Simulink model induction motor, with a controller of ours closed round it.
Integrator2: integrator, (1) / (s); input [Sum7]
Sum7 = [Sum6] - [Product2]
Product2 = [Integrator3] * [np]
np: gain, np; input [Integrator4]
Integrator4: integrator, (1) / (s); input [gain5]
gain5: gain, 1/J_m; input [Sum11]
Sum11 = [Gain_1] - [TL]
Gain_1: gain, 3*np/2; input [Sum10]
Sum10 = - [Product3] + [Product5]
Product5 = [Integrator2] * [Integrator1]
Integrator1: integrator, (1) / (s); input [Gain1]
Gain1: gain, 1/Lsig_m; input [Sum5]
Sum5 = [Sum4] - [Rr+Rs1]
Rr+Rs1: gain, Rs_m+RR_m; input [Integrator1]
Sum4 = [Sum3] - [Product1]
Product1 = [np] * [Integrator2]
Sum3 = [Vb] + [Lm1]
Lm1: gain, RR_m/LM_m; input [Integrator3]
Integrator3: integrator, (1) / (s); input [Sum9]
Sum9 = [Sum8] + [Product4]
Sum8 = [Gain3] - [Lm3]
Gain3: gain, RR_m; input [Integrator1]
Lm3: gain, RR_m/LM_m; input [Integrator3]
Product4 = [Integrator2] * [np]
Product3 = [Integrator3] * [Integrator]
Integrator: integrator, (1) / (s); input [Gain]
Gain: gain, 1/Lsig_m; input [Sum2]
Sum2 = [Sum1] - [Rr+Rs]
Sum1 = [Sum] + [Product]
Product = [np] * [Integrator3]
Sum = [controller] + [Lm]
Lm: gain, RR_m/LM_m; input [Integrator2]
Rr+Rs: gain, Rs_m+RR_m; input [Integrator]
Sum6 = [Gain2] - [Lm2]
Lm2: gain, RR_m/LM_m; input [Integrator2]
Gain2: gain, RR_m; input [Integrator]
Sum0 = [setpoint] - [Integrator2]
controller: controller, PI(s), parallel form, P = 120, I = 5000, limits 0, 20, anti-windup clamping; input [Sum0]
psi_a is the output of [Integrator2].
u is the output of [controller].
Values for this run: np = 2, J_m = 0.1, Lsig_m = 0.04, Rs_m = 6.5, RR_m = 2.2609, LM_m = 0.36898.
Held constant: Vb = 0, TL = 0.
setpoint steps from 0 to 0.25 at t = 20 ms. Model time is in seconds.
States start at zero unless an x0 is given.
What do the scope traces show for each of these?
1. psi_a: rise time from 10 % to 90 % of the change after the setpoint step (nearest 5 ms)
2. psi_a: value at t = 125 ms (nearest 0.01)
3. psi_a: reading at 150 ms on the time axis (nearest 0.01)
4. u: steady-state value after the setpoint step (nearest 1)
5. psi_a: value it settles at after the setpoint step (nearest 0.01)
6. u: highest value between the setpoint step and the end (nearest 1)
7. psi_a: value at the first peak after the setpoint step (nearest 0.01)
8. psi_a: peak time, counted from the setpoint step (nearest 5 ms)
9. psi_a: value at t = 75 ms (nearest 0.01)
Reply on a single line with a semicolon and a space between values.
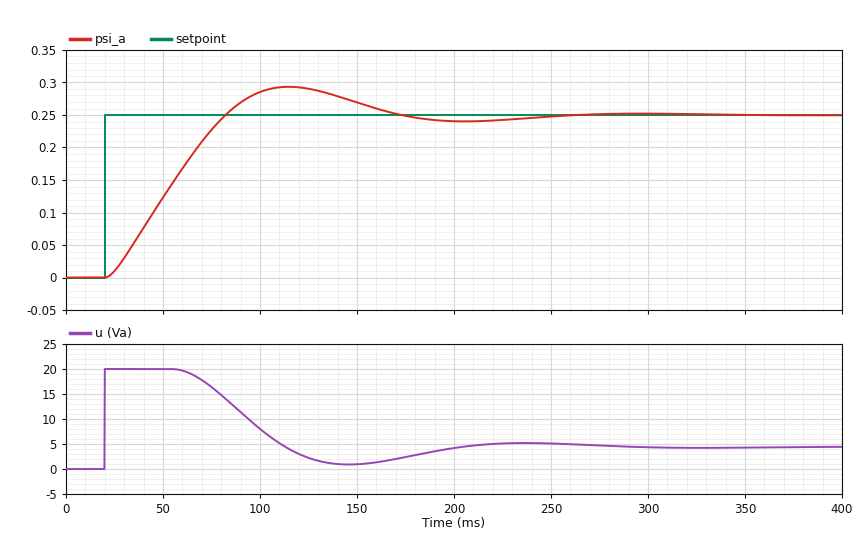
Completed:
45 ms; 0.29; 0.27; 4; 0.25; 20; 0.29; 95 ms; 0.23
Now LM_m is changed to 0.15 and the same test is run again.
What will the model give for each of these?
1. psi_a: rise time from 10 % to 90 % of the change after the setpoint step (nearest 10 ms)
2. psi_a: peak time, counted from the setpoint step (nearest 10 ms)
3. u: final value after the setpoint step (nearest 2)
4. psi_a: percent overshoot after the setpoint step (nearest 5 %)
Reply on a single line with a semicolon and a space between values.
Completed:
60 ms; 110 ms; 10; 10 %
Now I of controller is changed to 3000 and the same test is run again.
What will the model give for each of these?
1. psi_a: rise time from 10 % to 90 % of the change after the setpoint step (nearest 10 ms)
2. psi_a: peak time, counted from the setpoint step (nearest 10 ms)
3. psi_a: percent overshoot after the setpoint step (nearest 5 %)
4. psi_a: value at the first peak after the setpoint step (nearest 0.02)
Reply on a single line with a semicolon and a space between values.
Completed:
50 ms; 110 ms; 10 %; 0.28
